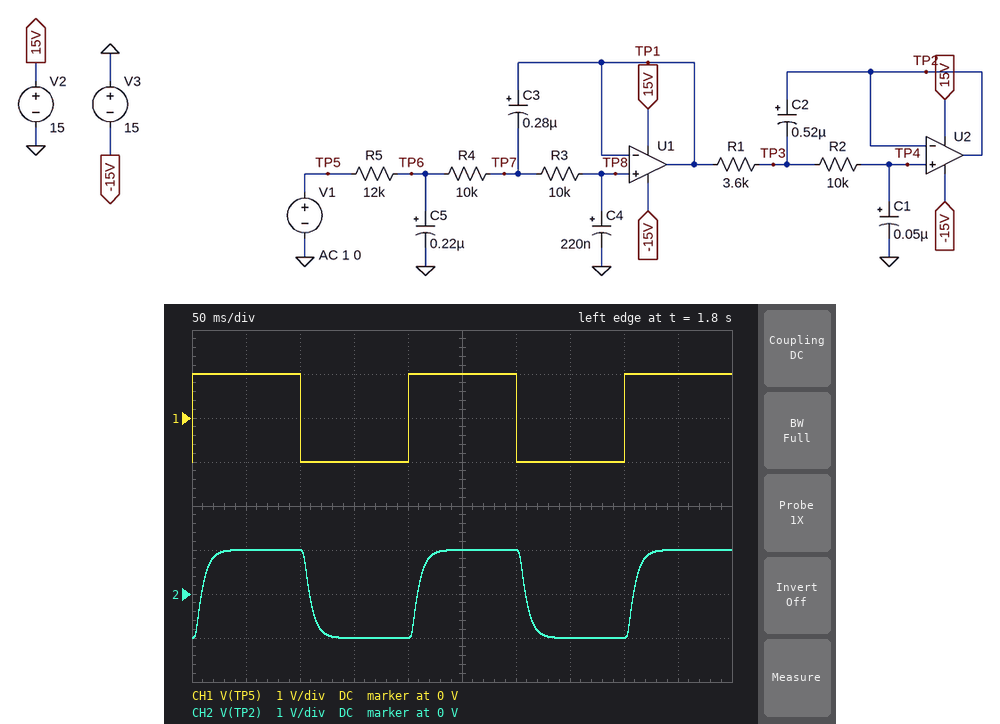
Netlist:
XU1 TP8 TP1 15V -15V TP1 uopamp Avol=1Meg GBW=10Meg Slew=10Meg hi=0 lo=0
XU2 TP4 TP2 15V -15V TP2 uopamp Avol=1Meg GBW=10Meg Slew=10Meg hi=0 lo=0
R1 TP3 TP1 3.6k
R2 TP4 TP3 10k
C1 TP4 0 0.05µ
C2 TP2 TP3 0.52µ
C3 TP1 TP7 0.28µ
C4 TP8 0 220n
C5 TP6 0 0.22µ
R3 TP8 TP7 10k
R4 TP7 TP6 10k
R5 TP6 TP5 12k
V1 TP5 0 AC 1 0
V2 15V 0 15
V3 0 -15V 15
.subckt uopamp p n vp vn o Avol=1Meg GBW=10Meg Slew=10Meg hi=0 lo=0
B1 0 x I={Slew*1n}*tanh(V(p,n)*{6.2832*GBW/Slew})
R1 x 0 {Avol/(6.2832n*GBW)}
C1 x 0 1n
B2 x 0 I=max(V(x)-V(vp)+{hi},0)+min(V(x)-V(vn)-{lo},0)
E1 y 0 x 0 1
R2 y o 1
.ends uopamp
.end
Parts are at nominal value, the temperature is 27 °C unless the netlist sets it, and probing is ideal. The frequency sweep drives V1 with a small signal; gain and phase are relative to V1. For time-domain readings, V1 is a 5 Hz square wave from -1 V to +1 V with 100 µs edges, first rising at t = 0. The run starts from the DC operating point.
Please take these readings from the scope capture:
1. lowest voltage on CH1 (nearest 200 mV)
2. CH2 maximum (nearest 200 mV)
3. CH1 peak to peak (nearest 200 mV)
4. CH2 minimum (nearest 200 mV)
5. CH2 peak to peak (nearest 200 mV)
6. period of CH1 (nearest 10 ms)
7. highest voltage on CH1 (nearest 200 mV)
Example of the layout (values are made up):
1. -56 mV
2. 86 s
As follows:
1. -1.0 V
2. 1.0 V
3. 2.0 V
4. -1.0 V
5. 2.0 V
6. 200 ms
7. 1.0 V
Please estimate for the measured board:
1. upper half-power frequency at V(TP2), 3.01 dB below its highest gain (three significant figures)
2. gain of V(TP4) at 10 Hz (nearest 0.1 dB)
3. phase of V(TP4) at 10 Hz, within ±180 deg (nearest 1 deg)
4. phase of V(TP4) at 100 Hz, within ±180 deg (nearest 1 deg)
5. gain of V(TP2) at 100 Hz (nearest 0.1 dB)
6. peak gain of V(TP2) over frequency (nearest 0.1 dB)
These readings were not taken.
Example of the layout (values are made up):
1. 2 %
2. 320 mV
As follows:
1. 23.1 Hz
2. -0.7 dB
3. -36 deg
4. 159 deg
5. -16.9 dB
6. 0 dB
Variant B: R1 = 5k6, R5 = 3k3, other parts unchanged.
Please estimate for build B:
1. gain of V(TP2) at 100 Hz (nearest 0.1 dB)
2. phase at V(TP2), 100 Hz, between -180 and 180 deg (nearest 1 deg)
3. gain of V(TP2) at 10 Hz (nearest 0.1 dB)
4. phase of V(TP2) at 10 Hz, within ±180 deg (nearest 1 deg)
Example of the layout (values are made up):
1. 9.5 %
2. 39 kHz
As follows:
1. -9.0 dB
2. 167 deg
3. -0.2 dB
4. -24 deg
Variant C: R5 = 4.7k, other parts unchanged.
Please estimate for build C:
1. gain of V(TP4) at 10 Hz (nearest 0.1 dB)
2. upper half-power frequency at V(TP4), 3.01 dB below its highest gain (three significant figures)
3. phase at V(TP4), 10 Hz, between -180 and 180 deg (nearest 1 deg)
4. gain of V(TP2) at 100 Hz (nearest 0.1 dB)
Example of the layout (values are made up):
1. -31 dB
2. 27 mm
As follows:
1. -0.2 dB
2. 37.9 Hz
3. -26 deg
4. -11.7 dB
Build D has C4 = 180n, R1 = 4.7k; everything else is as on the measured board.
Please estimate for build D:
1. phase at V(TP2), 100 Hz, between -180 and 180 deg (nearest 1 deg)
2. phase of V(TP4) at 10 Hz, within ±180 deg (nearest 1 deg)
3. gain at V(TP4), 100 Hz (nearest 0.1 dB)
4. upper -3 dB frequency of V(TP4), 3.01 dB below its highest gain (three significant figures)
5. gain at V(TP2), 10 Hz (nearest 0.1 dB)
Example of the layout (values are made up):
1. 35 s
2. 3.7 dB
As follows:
1. 154 deg
2. -32 deg
3. -14.2 dB
4. 28.2 Hz
5. -0.5 dB
